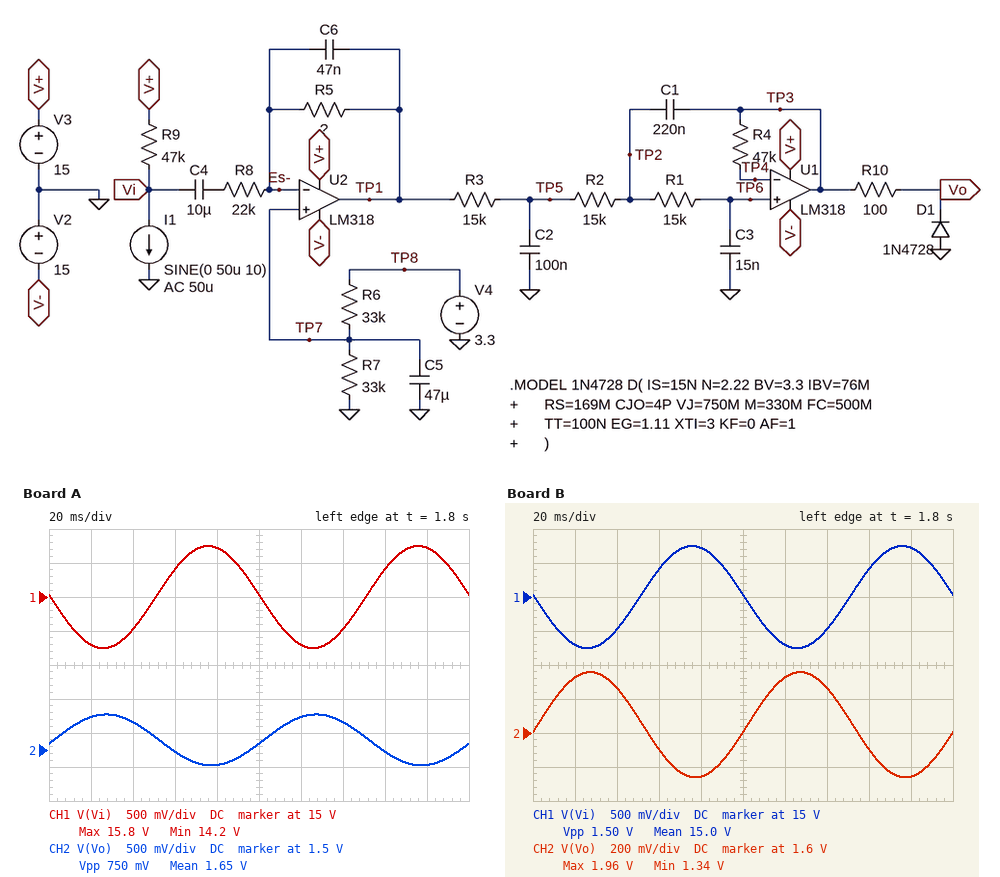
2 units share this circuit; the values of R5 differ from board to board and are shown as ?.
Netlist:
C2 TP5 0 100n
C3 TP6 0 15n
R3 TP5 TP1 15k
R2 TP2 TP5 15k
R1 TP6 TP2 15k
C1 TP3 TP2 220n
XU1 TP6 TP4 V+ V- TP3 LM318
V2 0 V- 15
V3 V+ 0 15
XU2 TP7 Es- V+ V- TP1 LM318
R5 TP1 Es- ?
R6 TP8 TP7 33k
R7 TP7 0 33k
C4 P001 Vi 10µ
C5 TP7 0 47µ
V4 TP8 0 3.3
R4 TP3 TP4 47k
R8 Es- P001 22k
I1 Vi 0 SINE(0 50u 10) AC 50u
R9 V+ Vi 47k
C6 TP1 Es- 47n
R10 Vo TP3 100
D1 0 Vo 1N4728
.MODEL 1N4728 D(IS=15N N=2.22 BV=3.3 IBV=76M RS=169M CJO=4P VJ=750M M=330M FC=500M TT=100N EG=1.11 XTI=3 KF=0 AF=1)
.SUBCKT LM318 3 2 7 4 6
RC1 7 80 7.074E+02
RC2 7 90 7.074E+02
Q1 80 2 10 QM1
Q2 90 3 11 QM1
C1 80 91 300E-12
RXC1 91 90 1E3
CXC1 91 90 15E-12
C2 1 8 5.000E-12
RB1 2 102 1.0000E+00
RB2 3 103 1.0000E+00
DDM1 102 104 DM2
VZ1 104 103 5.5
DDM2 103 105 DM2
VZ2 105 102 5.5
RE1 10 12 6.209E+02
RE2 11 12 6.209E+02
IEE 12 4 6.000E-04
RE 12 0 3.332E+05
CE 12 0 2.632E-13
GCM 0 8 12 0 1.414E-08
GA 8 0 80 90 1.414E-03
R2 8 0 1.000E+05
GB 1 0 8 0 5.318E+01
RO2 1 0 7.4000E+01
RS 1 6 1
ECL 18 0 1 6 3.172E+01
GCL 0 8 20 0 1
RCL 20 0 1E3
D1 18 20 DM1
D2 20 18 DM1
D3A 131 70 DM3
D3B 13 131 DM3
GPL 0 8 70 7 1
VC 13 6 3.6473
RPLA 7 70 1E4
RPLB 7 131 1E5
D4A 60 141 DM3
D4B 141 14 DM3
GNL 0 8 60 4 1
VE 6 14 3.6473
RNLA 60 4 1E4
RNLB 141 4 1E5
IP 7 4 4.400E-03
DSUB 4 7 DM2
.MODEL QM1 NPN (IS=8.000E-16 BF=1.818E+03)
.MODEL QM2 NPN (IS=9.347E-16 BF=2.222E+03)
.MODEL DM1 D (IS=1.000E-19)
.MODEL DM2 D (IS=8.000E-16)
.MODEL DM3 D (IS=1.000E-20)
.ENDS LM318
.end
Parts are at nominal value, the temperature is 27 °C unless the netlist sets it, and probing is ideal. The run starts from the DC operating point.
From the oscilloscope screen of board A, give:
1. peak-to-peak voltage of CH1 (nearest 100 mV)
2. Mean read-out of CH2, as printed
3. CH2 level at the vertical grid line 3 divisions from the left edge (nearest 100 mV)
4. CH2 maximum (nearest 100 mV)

1.5 V
1.65 V
1.5 V
2.0 V
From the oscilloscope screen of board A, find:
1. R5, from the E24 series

11 kΩ
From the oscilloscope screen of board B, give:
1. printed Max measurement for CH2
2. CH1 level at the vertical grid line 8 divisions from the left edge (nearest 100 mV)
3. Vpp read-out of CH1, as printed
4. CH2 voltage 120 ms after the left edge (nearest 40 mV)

1.96 V
15.4 V
1.50 V
1.92 V
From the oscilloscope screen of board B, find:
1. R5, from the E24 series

9.1 kΩ
